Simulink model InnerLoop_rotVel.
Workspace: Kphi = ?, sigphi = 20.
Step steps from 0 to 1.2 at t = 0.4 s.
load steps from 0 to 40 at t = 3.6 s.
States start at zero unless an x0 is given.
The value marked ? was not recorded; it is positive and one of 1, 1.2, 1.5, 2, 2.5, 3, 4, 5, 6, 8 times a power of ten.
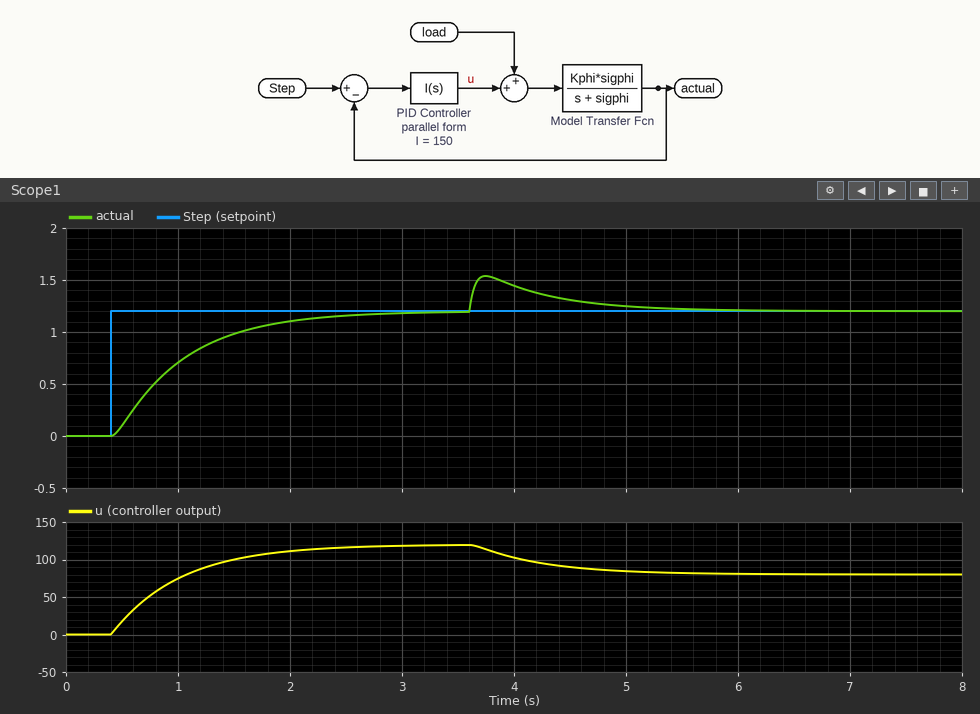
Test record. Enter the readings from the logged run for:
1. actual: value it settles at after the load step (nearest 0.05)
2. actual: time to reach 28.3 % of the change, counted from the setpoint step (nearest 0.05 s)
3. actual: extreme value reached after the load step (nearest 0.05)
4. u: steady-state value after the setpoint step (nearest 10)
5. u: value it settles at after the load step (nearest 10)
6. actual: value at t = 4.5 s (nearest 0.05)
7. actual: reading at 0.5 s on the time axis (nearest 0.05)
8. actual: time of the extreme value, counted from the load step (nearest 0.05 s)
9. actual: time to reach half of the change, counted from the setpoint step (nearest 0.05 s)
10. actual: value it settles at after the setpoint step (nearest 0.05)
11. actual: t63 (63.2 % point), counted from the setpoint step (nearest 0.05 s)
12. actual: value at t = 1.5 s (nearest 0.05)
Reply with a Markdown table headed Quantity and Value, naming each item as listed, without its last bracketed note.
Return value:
| Quantity | Value |
|---|---|
| actual: value it settles at after the load step | 1.20 |
| actual: time to reach 28.3 % of the change, counted from the setpoint step | 0.25 s |
| actual: extreme value reached after the load step | 1.55 |
| u: steady-state value after the setpoint step | 120 |
| u: value it settles at after the load step | 80 |
| actual: value at t = 4.5 s | 1.30 |
| actual: reading at 0.5 s on the time axis | 0.10 |
| actual: time of the extreme value, counted from the load step | 0.15 s |
| actual: time to reach half of the change, counted from the setpoint step | 0.50 s |
| actual: value it settles at after the setpoint step | 1.20 |
| actual: t63 (63.2 % point), counted from the setpoint step | 0.65 s |
| actual: value at t = 1.5 s | 1.00 |
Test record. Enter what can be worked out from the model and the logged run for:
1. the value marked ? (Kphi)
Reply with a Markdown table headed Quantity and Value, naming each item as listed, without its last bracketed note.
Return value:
| Quantity | Value |
|---|---|
| the value marked ? | 0.01 |
